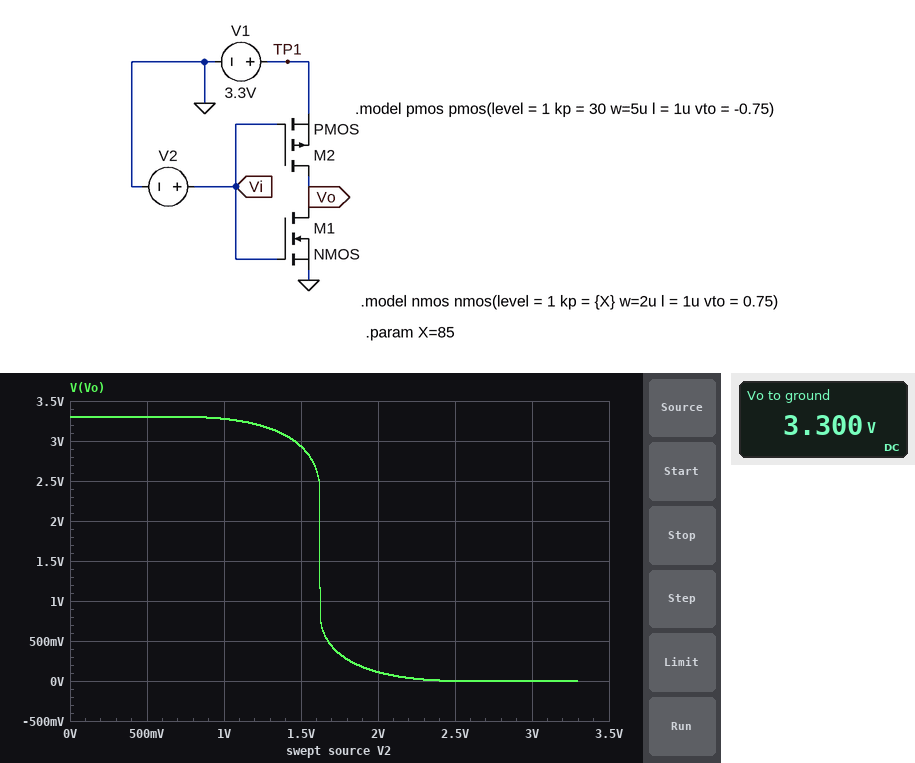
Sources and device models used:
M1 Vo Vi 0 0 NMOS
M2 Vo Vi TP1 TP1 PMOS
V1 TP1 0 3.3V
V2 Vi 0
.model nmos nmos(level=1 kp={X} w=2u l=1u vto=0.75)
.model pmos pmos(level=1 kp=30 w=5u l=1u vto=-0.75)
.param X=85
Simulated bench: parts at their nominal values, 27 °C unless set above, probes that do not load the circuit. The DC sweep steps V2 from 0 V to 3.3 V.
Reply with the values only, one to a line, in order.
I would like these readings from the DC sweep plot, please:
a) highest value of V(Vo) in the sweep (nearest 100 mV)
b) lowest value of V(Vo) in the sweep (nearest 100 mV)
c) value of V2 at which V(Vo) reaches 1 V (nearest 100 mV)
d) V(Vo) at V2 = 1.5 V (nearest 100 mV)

3.3 V
0 V
1.6 V
2.9 V
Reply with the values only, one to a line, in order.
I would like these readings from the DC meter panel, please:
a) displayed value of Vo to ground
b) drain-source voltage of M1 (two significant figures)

3.300 V
3.3 V
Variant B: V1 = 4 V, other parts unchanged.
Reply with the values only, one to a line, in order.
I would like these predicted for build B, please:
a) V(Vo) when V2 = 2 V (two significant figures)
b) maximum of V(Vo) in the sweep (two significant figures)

820 mV
4.0 V
